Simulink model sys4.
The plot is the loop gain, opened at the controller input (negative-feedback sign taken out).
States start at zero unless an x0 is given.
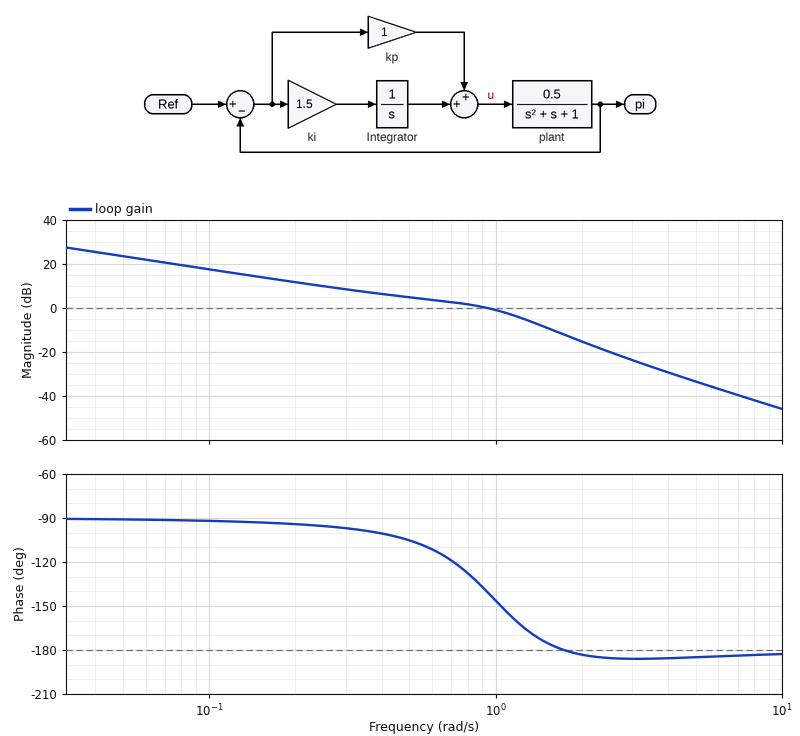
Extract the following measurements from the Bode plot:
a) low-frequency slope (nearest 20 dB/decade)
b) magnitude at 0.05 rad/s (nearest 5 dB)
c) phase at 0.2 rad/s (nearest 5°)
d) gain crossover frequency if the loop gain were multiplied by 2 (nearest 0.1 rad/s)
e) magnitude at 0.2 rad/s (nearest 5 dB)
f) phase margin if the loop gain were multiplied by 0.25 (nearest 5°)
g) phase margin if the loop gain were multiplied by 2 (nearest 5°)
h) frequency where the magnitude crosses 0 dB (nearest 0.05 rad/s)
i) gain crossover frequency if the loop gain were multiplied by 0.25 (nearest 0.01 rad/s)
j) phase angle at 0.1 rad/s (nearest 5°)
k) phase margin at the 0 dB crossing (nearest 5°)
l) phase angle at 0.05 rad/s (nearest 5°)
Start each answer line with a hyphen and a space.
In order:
- -20 dB/decade
- 25 dB
- -95°
- 1.3 rad/s
- 10 dB
- 85°
- 10°
- 0.95 rad/s
- 0.19 rad/s
- -90°
- 40°
- -90°
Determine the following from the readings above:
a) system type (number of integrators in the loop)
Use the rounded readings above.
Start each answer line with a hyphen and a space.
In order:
- 1
